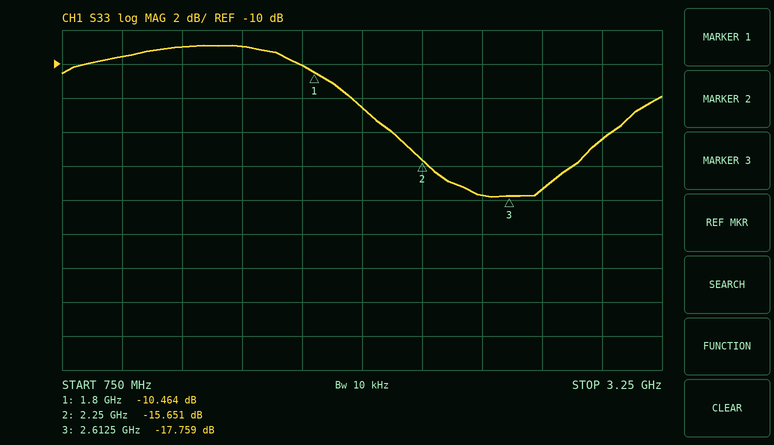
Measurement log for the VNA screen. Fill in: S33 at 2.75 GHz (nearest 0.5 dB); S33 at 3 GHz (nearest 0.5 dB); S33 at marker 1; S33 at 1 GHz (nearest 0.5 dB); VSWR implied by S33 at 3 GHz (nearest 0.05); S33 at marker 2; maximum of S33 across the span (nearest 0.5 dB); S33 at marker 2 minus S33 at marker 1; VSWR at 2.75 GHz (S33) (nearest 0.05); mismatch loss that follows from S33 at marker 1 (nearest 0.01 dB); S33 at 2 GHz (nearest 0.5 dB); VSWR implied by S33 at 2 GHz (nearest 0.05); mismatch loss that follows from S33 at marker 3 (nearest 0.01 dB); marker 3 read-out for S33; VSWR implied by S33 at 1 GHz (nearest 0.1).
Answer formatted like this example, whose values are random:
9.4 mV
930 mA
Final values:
-17.5 dB
-14.5 dB
-10.464 dB
-9.5 dB
1.45
-15.651 dB
-9.0 dB
-5.187 dB
1.30
0.41 dB
-12.5 dB
1.60
0.07 dB
-17.759 dB
2.0
